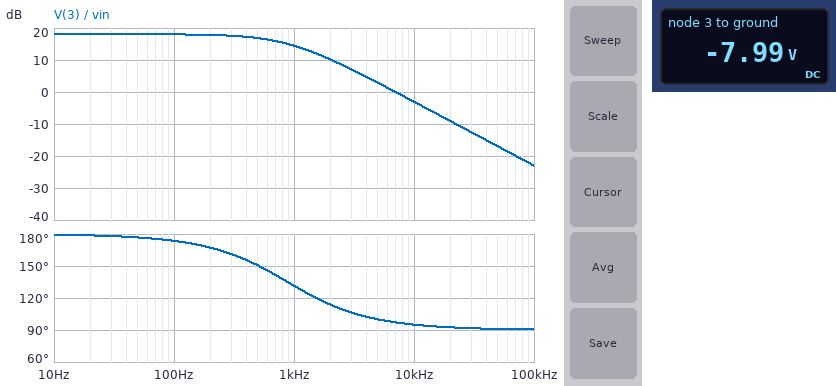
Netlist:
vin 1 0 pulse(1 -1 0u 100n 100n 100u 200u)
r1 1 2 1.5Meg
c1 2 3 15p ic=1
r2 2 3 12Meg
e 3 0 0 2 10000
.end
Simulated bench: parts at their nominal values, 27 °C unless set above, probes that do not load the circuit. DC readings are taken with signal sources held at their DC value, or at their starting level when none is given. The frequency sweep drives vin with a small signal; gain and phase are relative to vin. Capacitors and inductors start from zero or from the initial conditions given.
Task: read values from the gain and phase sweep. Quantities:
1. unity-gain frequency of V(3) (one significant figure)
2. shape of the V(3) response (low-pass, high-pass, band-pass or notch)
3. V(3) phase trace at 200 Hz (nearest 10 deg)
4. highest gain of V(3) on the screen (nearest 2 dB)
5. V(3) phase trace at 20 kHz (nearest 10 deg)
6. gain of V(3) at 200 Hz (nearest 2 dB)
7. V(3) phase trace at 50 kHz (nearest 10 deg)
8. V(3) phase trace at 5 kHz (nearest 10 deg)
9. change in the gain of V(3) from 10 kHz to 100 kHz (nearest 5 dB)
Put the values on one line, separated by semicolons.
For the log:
7 kHz; low-pass; 170 deg; 18 dB; 90 deg; 18 dB; 90 deg; 100 deg; -20 dB
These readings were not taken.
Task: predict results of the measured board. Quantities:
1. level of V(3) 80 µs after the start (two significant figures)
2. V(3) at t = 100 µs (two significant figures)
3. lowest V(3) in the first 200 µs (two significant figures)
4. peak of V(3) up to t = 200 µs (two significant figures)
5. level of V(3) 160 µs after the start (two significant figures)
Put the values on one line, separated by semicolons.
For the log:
2.2 V; 2.8 V; -1.8 V; 2.8 V; -230 mV
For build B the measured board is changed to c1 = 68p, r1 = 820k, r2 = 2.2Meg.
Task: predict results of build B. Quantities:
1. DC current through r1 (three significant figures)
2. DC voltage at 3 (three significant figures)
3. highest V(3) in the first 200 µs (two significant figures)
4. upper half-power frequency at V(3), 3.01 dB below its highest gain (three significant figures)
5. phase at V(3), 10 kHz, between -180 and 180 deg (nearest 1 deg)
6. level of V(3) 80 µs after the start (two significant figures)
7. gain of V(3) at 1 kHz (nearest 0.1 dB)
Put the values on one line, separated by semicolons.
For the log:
1.22 µA; -2.68 V; 800 mV; 1.06 kHz; 96 deg; 520 mV; 5.8 dB
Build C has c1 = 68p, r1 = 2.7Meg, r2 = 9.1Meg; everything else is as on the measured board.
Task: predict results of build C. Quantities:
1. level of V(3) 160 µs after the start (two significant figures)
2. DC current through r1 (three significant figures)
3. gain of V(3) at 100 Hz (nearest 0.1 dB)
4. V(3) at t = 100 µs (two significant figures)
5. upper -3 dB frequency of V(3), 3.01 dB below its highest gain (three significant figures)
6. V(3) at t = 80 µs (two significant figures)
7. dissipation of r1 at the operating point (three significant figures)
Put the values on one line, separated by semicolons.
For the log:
-630 mV; 370 nA; 9.9 dB; -350 mV; 257 Hz; -470 mV; 370 nW
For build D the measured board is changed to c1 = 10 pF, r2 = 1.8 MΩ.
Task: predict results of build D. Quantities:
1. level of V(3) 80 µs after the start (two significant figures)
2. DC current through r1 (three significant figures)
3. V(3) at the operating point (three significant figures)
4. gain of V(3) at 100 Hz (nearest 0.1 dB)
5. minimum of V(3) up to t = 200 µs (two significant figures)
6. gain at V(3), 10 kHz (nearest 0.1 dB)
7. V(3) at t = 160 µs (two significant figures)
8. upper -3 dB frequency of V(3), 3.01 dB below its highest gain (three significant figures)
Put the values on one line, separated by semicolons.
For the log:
1.2 V; 667 nA; -1.20 V; 1.6 dB; -1.2 V; -2.0 dB; -1.1 V; 8.84 kHz
